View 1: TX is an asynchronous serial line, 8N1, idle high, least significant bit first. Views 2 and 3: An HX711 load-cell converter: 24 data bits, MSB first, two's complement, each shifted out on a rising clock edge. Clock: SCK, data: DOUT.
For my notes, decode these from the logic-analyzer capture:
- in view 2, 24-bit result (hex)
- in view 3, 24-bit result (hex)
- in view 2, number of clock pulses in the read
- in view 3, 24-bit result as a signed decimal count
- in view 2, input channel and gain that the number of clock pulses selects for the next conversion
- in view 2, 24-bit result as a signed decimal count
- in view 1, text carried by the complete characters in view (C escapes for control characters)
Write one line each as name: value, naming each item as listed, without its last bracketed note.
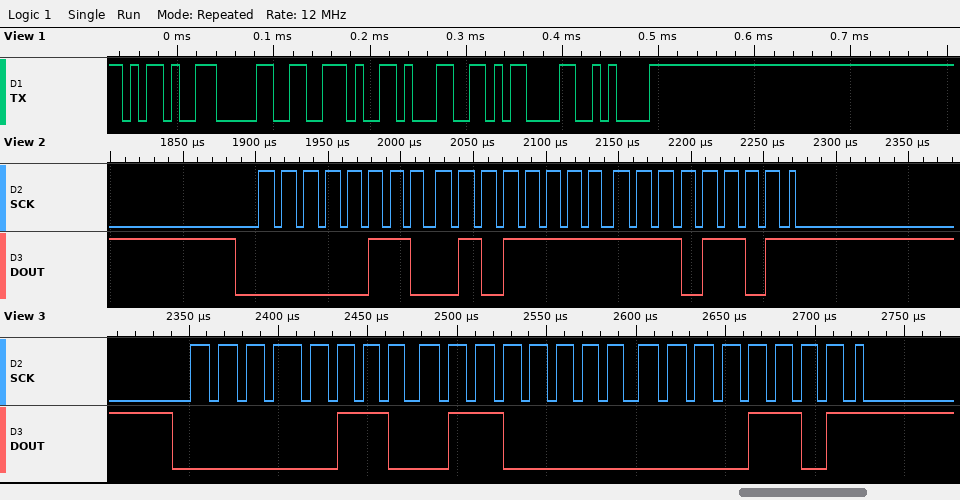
in view 2, 24-bit result: 0x065FED
in view 3, 24-bit result: 0x06600D
in view 2, number of clock pulses in the read: 25
in view 3, 24-bit result as a signed decimal count: 417805
in view 2, input channel and gain that the number of clock pulses selects for the next conversion: channel A, gain 128
in view 2, 24-bit result as a signed decimal count: 417773
in view 1, text carried by the complete characters in view: "-0.1\r\n"
